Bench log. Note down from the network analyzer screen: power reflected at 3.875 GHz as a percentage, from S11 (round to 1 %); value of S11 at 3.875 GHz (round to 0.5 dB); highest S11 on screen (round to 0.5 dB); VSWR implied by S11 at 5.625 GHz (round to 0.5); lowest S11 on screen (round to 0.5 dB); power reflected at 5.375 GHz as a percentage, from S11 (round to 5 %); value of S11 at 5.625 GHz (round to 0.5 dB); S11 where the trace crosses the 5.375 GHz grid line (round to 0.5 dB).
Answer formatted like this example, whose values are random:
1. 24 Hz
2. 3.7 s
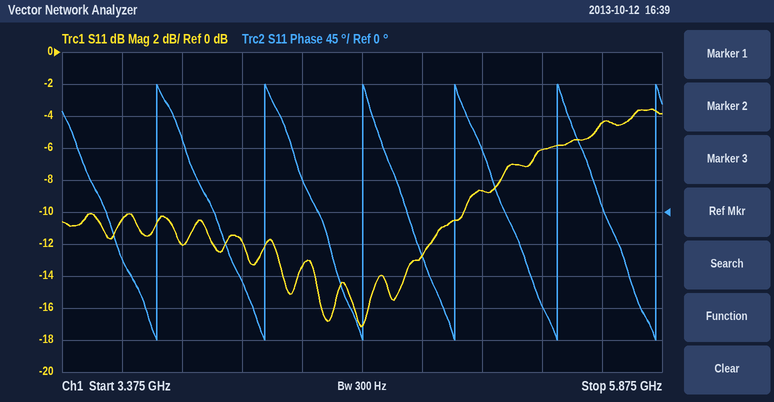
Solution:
1. 6 %
2. -12.0 dB
3. -3.5 dB
4. 4.0
5. -17.0 dB
6. 25 %
7. -4.5 dB
8. -6.0 dB
